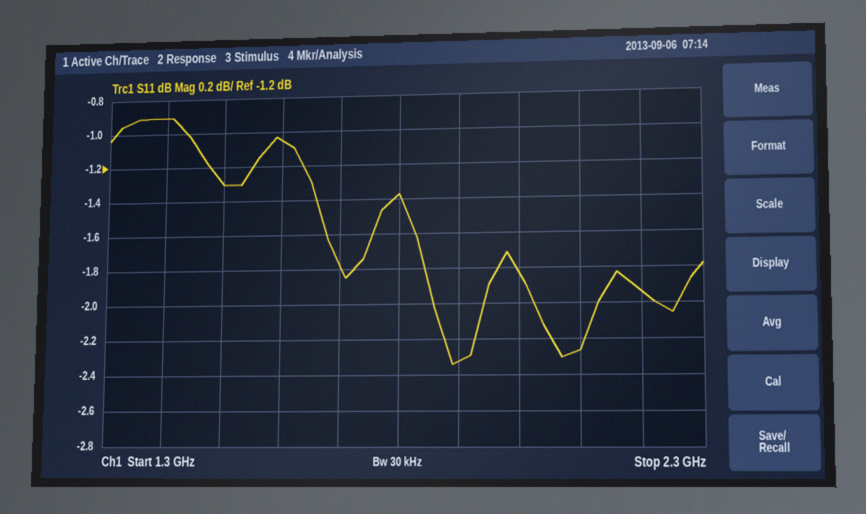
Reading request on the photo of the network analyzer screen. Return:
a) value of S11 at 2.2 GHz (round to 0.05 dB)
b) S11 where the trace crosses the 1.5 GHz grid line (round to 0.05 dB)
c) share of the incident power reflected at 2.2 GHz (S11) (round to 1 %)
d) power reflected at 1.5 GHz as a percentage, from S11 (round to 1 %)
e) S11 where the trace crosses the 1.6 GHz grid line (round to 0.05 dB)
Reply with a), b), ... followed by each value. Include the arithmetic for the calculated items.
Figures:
a) -1.95 dB
b) -1.30 dB
c) 10^(-1.95/10) ≈ 64 %
d) 10^(-1.3/10) ≈ 74 %
e) -1.05 dB
